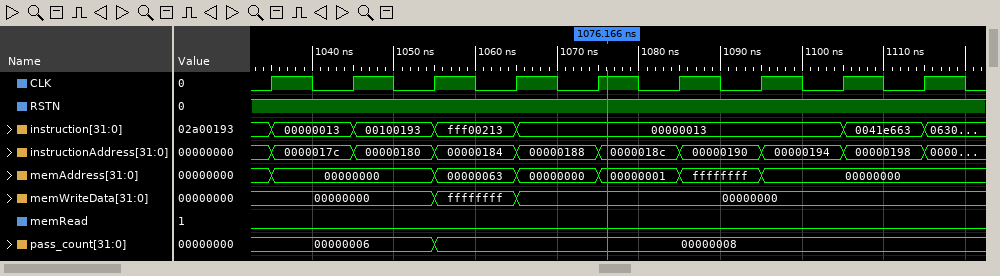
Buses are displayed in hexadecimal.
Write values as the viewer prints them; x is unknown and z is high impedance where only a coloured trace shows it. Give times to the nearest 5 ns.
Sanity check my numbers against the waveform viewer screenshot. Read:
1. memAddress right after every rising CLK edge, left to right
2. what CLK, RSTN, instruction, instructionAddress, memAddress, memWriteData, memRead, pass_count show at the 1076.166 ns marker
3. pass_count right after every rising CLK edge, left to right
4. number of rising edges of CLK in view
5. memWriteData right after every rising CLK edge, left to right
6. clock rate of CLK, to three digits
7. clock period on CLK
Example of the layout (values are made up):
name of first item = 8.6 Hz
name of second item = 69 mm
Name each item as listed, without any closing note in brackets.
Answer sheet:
memAddress right after every rising CLK edge, left to right = 00000000, 00000000, 00000063, 00000000, 00000001, ffffffff, 00000000, 00000000, 00000000
what CLK, RSTN, instruction, instructionAddress, memAddress, memWriteData, memRead, pass_count show at the 1076.166 ns marker = CLK=1, RSTN=1, instruction=00000013, instructionAddress=0000018c, memAddress=00000001, memWriteData=00000000, memRead=0, pass_count=00000008
pass_count right after every rising CLK edge, left to right = 00000006, 00000006, 00000008, 00000008, 00000008, 00000008, 00000008, 00000008, 00000008
number of rising edges of CLK in view = 9
memWriteData right after every rising CLK edge, left to right = 00000000, 00000000, ffffffff, 00000000, 00000000, 00000000, 00000000, 00000000, 00000000
clock rate of CLK, to three digits = 100 MHz
clock period on CLK = 10 ns
